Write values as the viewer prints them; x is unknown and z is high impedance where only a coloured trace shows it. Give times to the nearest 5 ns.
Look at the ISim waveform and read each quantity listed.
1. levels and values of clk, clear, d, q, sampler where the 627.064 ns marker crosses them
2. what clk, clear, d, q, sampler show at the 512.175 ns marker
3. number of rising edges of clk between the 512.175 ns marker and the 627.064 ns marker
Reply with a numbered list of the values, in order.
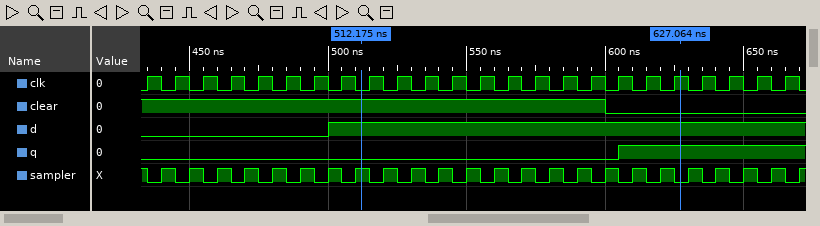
1. clk=1, clear=0, d=1, q=1, sampler=0
2. clk=0, clear=1, d=1, q=0, sampler=1
3. 12
